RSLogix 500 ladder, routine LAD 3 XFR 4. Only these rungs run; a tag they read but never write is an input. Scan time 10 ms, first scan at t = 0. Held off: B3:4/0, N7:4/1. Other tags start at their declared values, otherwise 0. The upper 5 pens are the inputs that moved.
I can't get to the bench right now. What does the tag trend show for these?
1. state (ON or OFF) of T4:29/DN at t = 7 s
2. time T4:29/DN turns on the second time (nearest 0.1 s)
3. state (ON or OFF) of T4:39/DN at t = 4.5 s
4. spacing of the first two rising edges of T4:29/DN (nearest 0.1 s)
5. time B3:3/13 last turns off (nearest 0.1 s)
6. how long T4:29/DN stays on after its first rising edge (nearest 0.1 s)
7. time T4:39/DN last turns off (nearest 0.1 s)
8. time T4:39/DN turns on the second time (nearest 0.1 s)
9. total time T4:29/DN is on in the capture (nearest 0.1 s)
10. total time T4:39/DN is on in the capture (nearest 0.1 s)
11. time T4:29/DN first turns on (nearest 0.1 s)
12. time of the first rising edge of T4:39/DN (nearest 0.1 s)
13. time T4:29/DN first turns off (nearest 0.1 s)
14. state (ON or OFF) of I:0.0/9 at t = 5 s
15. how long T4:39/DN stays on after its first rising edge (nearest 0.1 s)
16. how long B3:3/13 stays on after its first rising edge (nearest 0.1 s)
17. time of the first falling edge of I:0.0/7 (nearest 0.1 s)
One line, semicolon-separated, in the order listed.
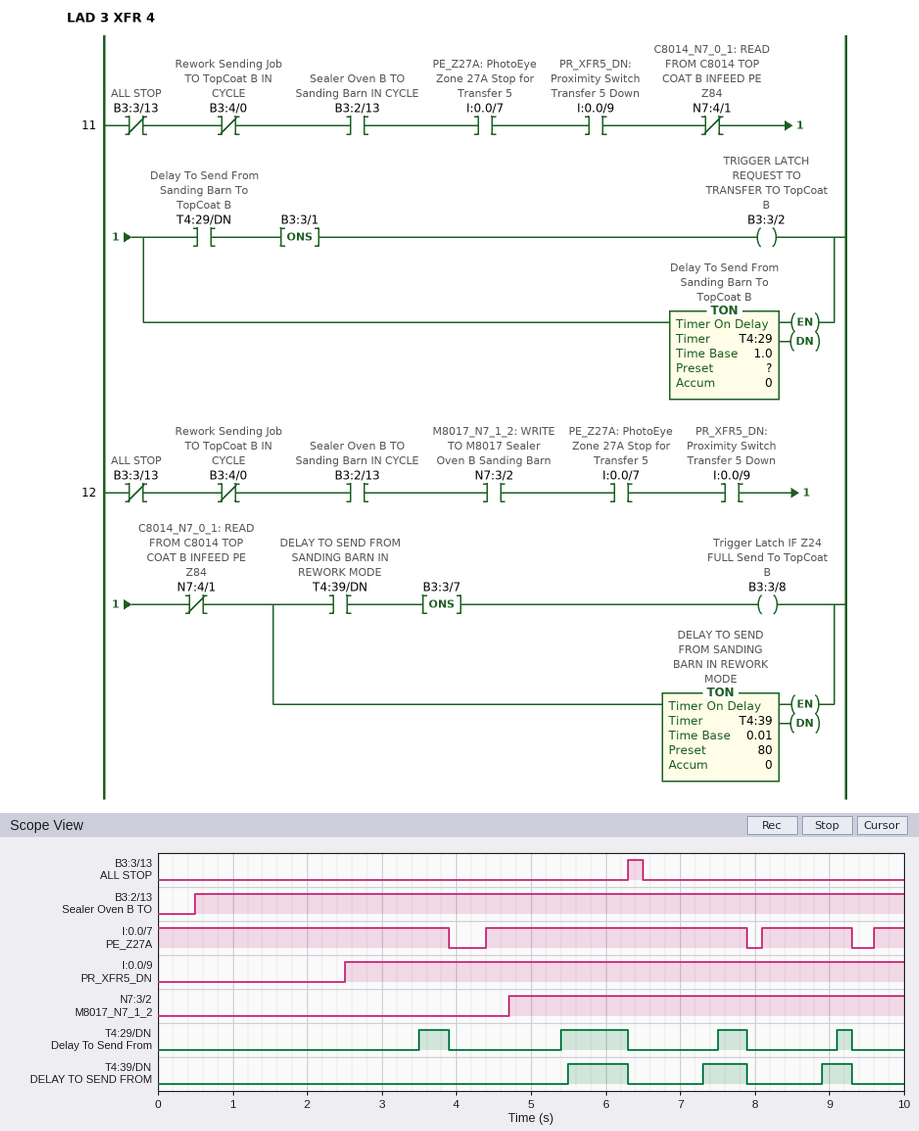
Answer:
OFF; 5.4 s; OFF; 1.9 s; 6.5 s; 0.4 s; 9.3 s; 7.3 s; 1.9 s; 1.8 s; 3.5 s; 5.5 s; 3.9 s; ON; 0.8 s; 0.2 s; 3.9 s
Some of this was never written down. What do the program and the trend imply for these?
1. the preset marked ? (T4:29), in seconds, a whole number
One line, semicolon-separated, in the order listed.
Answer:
1 s
